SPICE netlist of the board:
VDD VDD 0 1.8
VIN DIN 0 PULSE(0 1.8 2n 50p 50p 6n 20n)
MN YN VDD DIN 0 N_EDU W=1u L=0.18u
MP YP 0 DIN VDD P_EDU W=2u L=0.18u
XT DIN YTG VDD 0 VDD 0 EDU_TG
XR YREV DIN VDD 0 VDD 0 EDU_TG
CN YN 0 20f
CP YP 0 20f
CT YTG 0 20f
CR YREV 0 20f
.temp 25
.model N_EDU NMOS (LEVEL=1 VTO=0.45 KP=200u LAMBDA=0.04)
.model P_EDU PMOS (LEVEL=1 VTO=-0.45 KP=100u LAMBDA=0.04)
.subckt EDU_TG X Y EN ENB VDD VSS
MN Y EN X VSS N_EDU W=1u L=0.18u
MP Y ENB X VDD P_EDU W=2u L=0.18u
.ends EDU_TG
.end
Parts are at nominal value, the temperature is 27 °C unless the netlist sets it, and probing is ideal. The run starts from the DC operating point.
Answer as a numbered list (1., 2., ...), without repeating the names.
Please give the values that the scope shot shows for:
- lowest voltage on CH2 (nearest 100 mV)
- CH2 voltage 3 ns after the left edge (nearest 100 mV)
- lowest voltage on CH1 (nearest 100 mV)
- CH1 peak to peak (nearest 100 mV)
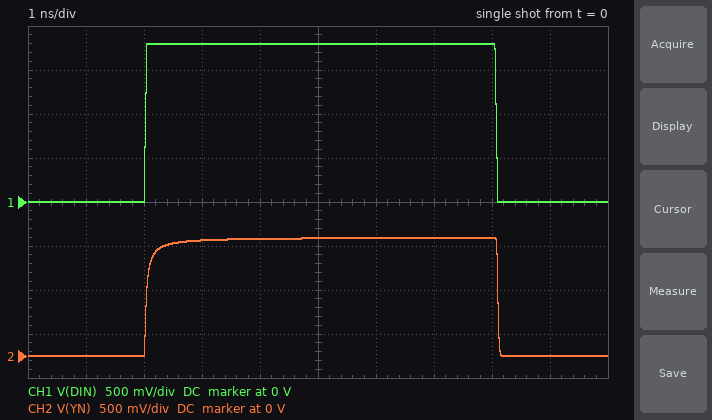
1. 0 V
2. 1.3 V
3. 0 V
4. 1.8 V
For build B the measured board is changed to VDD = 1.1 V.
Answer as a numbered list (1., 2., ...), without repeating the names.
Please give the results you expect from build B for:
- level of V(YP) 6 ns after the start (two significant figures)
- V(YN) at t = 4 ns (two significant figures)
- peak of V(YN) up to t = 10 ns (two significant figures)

1. 1.7 V
2. 630 mV
3. 640 mV
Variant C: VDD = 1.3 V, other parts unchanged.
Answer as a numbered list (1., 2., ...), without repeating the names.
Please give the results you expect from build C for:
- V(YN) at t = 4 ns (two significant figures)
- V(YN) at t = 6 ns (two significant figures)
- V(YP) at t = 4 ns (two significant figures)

1. 830 mV
2. 840 mV
3. 1.8 V
